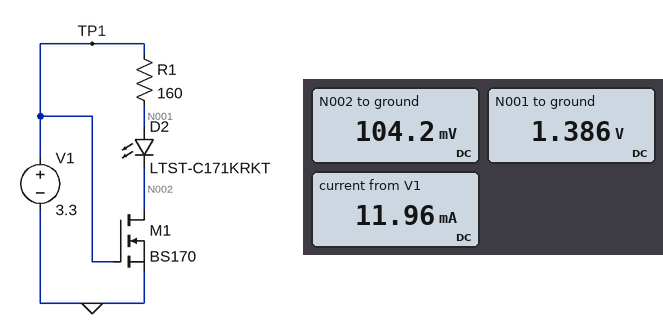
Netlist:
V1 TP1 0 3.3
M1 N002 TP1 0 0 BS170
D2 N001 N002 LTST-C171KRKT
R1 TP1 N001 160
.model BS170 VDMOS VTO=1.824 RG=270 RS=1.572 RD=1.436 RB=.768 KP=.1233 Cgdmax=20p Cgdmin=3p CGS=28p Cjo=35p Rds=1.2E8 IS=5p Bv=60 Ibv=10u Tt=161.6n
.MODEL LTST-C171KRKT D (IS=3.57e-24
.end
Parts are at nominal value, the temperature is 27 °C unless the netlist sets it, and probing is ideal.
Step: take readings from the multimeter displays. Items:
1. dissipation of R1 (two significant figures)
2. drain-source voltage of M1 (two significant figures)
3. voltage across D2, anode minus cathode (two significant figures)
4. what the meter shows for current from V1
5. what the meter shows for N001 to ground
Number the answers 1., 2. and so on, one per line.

1. 23 mW
2. 100 mV
3. 1.3 V
4. 11.96 mA
5. 1.386 V
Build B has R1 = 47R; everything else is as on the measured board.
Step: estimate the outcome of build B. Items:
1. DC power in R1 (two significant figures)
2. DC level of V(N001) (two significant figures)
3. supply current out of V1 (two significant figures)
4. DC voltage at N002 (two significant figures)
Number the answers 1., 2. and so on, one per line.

1. 59 mW
2. 1.6 V
3. 35 mA
4. 330 mV
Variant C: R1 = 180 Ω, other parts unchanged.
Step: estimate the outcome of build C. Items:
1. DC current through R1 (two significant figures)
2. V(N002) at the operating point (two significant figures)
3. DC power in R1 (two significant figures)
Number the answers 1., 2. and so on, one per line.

1. 11 mA
2. 93 mV
3. 21 mW
